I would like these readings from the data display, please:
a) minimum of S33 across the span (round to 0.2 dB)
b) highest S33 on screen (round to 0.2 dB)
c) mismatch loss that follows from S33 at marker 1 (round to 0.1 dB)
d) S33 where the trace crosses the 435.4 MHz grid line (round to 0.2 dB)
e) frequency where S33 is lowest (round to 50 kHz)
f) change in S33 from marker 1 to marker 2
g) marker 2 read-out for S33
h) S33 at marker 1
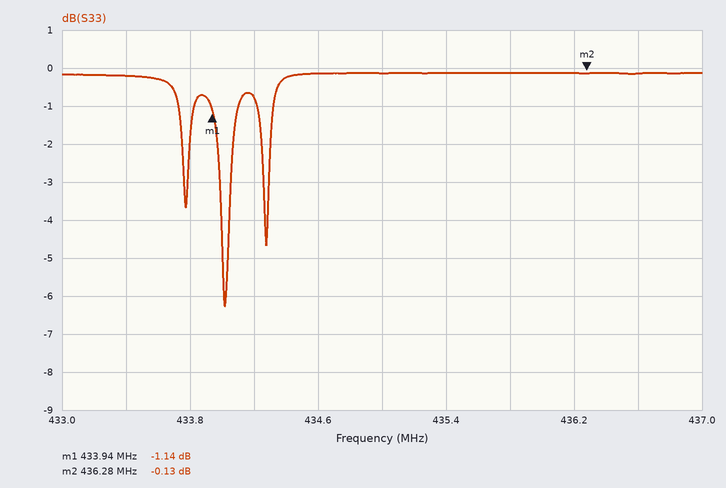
-6.2 dB
-0.2 dB
6.4 dB
-0.2 dB
434.00 MHz
1.01 dB
-0.13 dB
-1.14 dB
